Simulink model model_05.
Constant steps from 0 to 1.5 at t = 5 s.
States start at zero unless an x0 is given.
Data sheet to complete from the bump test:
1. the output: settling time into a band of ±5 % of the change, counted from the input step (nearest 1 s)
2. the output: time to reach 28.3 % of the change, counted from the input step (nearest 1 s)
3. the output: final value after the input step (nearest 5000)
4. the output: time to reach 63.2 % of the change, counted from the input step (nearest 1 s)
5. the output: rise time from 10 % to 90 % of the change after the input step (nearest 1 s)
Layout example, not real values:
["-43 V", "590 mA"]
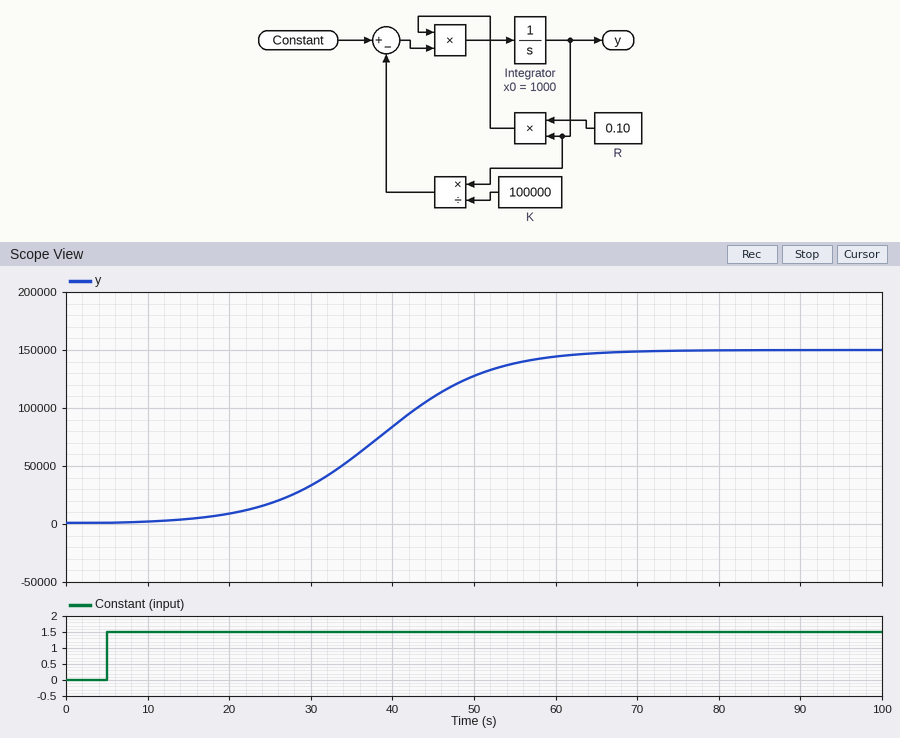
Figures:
["53 s", "27 s", "150000", "37 s", "29 s"]
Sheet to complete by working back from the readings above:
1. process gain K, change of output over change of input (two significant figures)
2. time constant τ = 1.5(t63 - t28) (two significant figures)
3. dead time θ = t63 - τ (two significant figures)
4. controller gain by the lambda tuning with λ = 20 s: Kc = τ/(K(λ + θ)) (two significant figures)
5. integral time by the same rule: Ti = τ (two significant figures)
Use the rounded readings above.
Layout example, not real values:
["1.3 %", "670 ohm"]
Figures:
["100000", "15 s", "22 s", "0.0000036", "15 s"]
